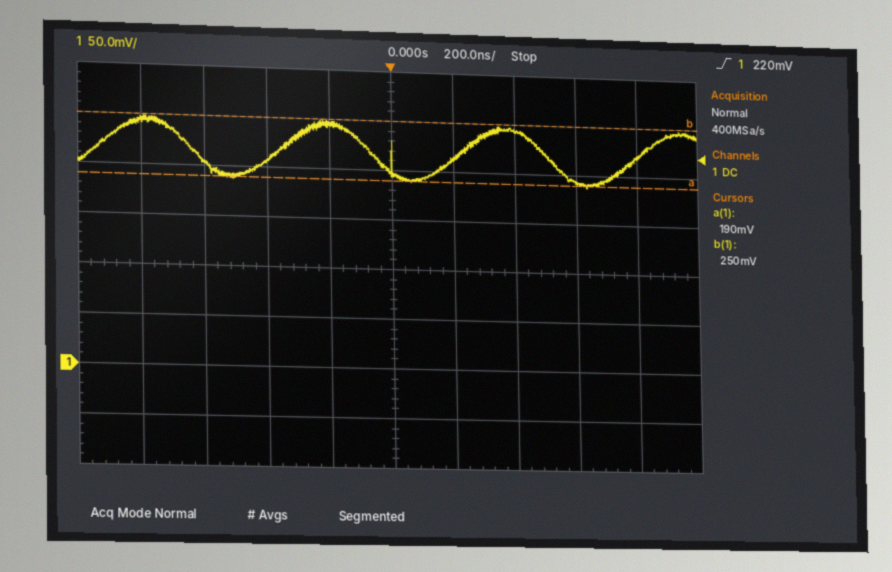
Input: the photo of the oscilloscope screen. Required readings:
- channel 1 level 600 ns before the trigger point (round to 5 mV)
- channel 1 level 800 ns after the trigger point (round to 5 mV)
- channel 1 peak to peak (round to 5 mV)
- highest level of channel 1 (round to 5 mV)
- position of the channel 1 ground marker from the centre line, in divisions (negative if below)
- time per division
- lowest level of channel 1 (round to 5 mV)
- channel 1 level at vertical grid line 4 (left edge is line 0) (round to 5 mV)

205 mV
220 mV
60 mV
250 mV
-2.0 div
200 ns
190 mV
245 mV
